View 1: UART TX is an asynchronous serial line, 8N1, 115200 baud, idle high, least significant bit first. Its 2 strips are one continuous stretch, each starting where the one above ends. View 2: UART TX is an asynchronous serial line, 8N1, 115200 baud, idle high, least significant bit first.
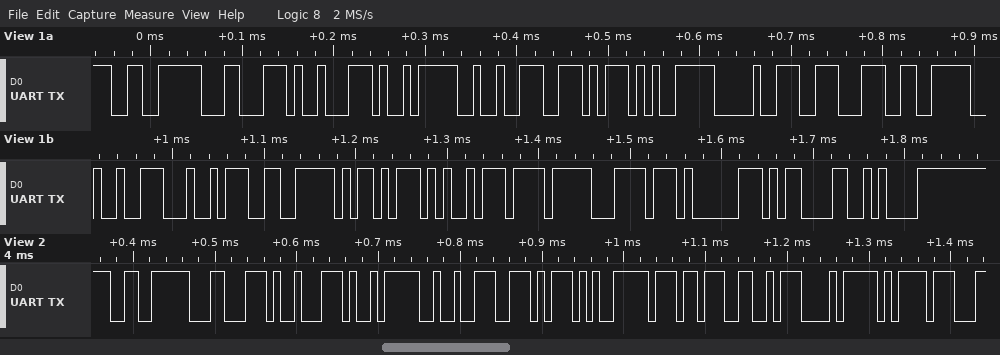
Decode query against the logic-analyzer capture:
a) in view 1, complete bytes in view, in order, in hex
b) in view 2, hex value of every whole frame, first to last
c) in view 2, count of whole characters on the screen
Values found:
E6 8C 89 E9 92 AE E5 90 8E E6 92 A4 E6 AD A5 EF BC 81 0D 0A
E6 8C 89 E9 92 AE E5 B7 A6 E8 BD
11
